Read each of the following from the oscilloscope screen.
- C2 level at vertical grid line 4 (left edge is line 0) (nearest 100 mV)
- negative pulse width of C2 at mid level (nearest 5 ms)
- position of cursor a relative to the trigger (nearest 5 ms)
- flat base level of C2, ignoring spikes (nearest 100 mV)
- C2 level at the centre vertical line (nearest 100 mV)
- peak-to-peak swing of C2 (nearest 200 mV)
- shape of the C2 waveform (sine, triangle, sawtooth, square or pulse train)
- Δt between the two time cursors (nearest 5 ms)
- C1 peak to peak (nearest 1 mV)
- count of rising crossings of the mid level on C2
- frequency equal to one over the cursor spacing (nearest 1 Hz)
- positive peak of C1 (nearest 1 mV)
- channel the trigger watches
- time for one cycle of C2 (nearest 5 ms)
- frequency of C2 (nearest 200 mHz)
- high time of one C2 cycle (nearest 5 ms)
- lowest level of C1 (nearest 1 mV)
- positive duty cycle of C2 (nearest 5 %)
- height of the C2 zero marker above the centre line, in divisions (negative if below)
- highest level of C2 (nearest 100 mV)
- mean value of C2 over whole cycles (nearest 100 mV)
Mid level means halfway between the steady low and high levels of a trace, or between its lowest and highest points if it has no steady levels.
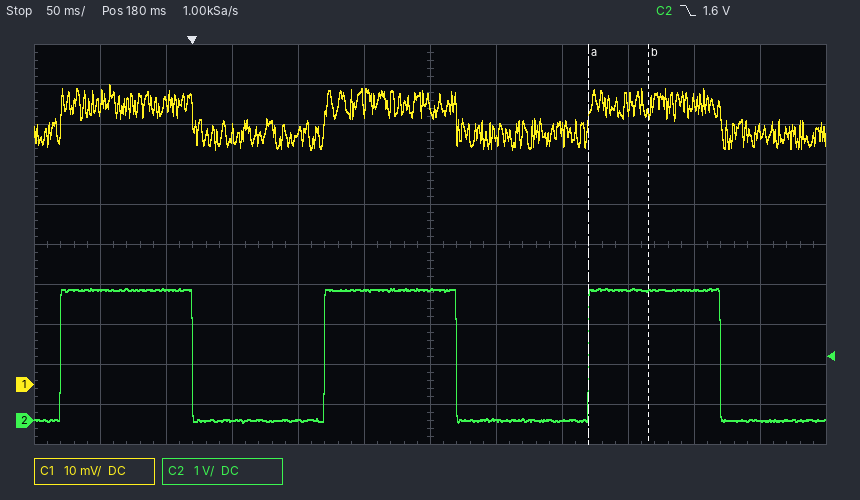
0.0 V
100 ms
+300 ms
0.0 V
3.3 V
3.4 V
square
45 ms
16 mV
3
22 Hz
75 mV
C2
200 ms
5.0 Hz
100 ms
59 mV
50 %
-4.4 div
3.3 V
1.6 V
